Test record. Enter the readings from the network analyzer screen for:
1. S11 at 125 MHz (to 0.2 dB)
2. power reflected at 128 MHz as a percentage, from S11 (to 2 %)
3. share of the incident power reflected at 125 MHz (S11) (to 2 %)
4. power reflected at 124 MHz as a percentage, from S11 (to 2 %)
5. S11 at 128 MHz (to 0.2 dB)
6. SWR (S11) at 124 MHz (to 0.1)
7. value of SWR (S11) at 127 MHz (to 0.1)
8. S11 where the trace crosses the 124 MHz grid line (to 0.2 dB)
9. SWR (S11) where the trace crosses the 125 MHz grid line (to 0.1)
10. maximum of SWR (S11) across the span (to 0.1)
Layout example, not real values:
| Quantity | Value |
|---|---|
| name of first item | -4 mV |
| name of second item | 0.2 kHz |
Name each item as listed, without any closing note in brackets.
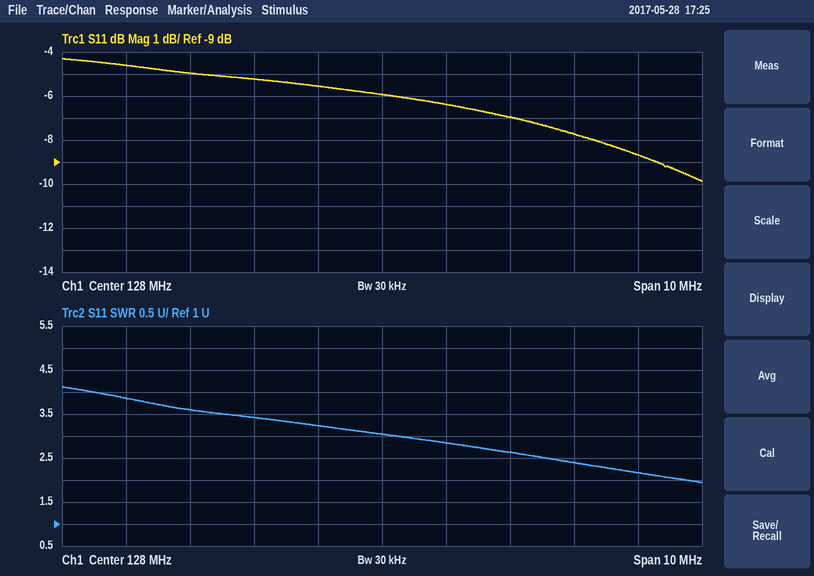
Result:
| Quantity | Value |
|---|---|
| S11 at 125 MHz | -5.0 dB |
| power reflected at 128 MHz as a percentage, from S11 | 26 % |
| share of the incident power reflected at 125 MHz (S11) | 32 % |
| power reflected at 124 MHz as a percentage, from S11 | 34 % |
| S11 at 128 MHz | -6.0 dB |
| SWR (S11) at 124 MHz | 3.9 |
| value of SWR (S11) at 127 MHz | 3.2 |
| S11 where the trace crosses the 124 MHz grid line | -4.6 dB |
| SWR (S11) where the trace crosses the 125 MHz grid line | 3.6 |
| maximum of SWR (S11) across the span | 4.1 |
